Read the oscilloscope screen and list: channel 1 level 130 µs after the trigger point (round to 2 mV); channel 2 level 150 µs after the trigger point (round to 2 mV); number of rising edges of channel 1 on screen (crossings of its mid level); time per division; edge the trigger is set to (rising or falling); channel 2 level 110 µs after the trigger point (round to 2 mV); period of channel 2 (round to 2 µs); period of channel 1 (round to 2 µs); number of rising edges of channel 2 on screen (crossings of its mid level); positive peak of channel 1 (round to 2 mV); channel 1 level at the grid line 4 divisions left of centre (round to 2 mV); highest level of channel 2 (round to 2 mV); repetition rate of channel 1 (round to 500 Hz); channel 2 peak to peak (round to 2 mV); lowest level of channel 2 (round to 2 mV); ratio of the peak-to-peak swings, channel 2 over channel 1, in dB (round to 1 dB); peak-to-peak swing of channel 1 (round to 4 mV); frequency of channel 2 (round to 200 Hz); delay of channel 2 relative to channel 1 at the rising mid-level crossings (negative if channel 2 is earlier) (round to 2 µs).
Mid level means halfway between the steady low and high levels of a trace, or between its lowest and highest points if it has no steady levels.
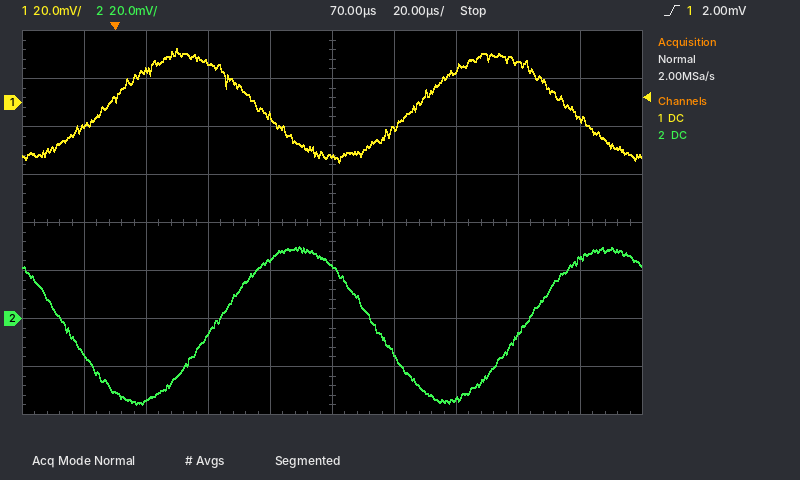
16 mV
24 mV
2
20 µs
rising
-34 mV
100 µs
100 µs
2
22 mV
-10 mV
30 mV
10.0 kHz
66 mV
-36 mV
3 dB
48 mV
10.0 kHz
+34 µs
